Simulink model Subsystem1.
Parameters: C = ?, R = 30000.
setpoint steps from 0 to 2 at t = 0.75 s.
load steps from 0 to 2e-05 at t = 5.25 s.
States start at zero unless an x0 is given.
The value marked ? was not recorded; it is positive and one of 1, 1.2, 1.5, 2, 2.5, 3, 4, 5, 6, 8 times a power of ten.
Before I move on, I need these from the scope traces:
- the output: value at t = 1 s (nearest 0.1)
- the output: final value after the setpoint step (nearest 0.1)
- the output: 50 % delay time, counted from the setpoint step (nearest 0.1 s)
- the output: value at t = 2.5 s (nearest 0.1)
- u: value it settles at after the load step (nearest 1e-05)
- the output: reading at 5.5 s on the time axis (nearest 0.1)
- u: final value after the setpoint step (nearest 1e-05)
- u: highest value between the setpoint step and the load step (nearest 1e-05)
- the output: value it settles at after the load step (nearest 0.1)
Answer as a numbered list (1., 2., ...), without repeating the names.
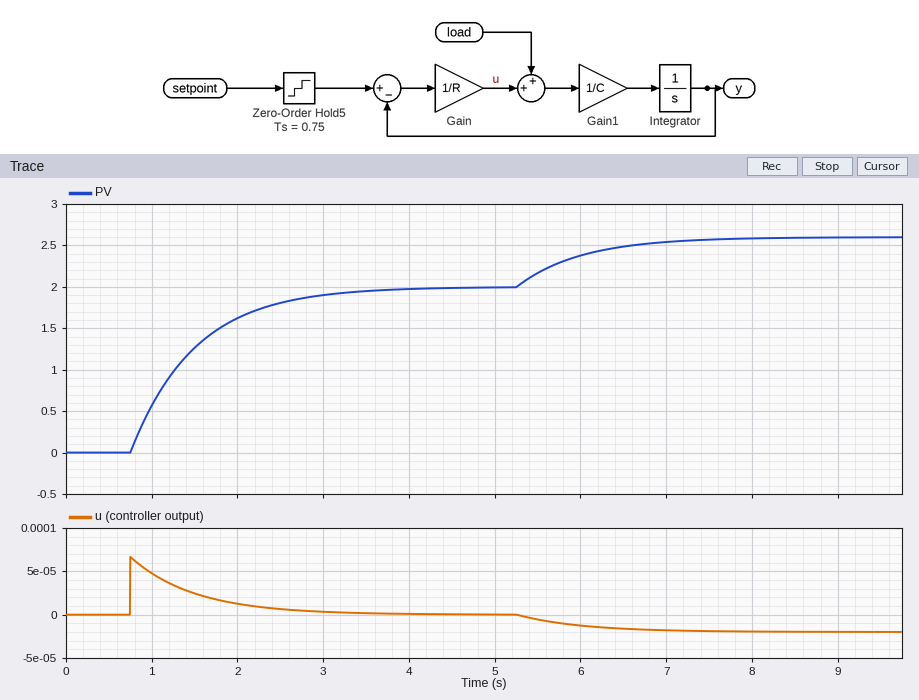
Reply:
1. 0.6
2. 2.0
3. 0.5 s
4. 1.8
5. -0.00002
6. 2.2
7. 0.00000
8. 0.00007
9. 2.6
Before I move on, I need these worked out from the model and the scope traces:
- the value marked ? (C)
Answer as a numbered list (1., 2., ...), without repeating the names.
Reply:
1. 2.5e-05
